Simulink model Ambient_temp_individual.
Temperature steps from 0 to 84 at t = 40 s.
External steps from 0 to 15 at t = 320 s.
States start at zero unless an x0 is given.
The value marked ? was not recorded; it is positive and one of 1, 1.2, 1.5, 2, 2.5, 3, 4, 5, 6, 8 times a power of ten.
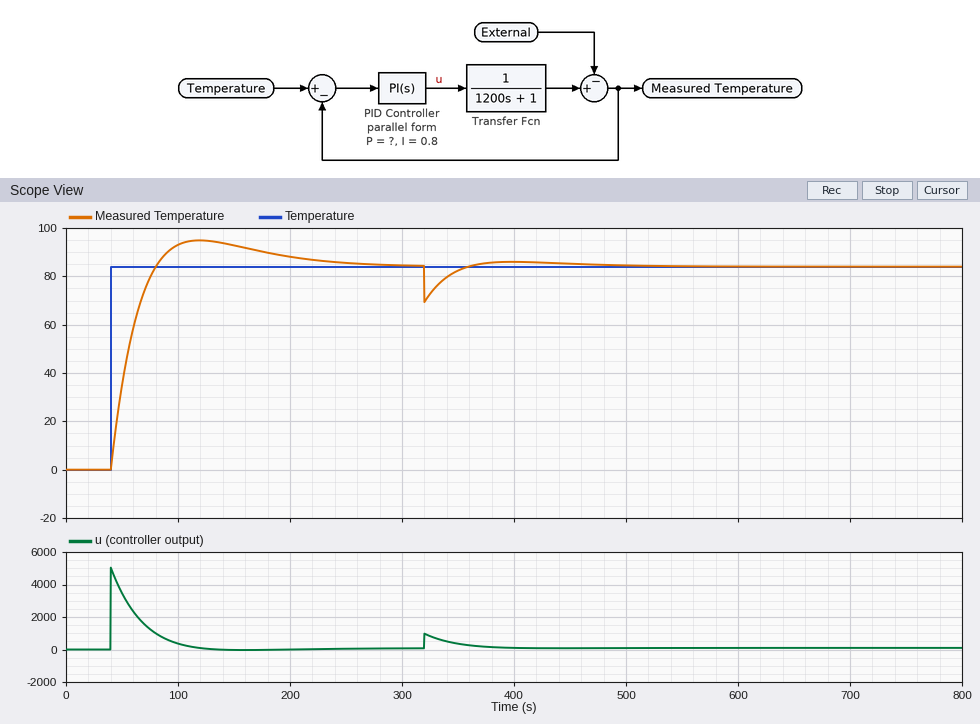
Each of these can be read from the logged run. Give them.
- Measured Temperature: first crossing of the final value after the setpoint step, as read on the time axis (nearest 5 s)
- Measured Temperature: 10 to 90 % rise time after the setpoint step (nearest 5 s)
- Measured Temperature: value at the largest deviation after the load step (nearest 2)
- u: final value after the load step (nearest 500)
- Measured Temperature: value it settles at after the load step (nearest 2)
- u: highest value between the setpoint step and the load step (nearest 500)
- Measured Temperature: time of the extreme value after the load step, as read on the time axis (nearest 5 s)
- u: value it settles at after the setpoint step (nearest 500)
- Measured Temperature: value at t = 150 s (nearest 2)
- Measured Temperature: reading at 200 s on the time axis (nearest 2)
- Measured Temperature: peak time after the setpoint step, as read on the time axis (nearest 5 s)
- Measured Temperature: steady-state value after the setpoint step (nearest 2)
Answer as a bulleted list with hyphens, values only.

- 80 s
- 30 s
- 70
- 0
- 84
- 5000
- 320 s
- 0
- 92
- 88
- 120 s
- 84
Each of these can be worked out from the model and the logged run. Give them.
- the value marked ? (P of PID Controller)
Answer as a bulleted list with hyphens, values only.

- 60
